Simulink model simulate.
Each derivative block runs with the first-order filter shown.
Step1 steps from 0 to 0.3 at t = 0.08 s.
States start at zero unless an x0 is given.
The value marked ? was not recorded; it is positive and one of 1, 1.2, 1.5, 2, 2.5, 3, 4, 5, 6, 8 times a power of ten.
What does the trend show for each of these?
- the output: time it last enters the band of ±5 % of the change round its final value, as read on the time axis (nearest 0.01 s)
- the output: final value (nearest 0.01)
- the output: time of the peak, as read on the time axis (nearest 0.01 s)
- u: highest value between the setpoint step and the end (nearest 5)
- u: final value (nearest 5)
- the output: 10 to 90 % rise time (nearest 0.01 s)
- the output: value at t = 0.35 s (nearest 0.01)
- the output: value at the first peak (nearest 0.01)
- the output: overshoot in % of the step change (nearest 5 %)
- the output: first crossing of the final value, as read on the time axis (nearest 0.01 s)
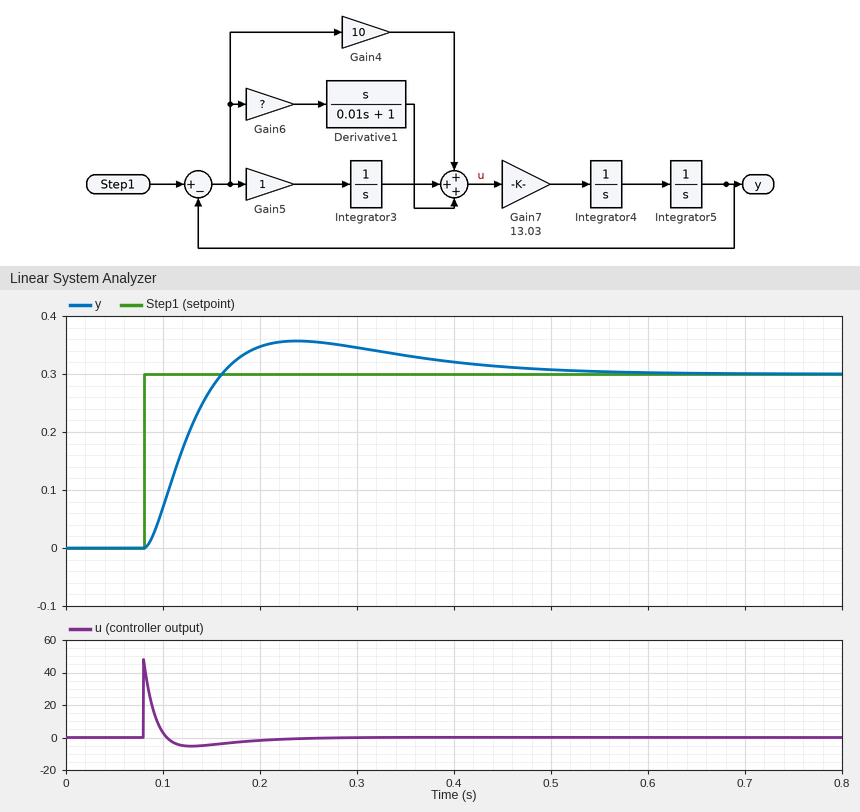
0.43 s
0.30
0.24 s
50
0
0.06 s
0.33
0.36
20 %
0.16 s
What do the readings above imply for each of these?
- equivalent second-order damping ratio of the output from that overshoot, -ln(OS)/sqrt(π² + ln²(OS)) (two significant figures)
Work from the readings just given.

0.46
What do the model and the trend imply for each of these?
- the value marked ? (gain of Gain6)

1.5
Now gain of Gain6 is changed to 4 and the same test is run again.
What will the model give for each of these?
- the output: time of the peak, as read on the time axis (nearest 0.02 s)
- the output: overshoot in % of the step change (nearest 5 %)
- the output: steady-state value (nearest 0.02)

0.14 s
10 %
0.30
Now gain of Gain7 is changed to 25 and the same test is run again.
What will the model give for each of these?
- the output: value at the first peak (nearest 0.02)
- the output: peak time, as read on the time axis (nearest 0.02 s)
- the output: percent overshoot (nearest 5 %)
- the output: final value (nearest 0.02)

0.34
0.16 s
15 %
0.30
